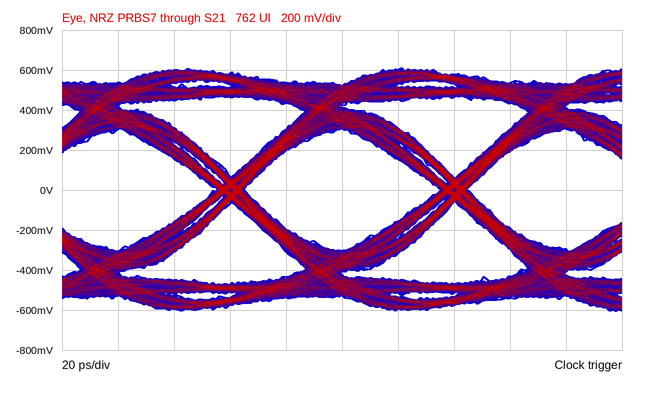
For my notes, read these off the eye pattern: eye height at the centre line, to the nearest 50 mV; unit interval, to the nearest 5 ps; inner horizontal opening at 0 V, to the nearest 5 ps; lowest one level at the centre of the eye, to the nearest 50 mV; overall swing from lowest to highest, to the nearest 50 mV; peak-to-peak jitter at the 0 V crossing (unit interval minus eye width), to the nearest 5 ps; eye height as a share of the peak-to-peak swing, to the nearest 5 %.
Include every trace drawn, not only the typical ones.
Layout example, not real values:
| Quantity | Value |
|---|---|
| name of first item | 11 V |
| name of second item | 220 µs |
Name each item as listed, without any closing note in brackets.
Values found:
| Quantity | Value |
|---|---|
| eye height at the centre line, to the nearest 50 mV | 600 mV |
| unit interval, to the nearest 5 ps | 80 ps |
| inner horizontal opening at 0 V, to the nearest 5 ps | 70 ps |
| lowest one level at the centre of the eye, to the nearest 50 mV | 300 mV |
| overall swing from lowest to highest, to the nearest 50 mV | 1.20 V |
| peak-to-peak jitter at the 0 V crossing (unit interval minus eye width), to the nearest 5 ps | 10 ps |
| eye height as a share of the peak-to-peak swing, to the nearest 5 % | 50 % |
